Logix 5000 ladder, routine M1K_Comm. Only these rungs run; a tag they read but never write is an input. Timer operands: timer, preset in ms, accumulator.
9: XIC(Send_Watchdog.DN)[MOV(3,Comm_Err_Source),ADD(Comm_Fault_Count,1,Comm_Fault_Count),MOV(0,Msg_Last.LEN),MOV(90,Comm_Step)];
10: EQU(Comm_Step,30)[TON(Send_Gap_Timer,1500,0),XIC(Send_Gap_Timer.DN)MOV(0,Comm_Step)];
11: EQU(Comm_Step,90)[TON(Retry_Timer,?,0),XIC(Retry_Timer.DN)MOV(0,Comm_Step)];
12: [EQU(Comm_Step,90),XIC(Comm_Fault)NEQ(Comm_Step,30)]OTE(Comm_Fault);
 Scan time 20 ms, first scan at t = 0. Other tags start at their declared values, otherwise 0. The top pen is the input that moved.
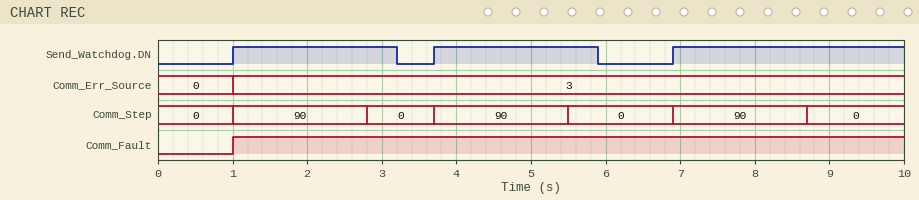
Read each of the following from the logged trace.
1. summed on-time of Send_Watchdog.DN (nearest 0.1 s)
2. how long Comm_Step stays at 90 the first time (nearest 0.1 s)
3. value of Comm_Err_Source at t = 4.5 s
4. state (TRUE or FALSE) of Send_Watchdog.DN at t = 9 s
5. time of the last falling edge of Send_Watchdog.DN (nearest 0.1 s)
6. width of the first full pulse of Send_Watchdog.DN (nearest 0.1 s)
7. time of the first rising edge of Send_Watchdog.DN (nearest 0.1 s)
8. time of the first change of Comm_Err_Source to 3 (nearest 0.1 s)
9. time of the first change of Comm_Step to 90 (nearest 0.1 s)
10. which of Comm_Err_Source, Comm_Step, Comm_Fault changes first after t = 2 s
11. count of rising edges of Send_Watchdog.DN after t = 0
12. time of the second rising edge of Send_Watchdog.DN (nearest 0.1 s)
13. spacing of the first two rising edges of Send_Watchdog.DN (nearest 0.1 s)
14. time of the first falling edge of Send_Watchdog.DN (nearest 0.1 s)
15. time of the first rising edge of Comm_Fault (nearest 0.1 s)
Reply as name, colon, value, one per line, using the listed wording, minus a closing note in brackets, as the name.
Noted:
summed on-time of Send_Watchdog.DN: 7.5 s
how long Comm_Step stays at 90 the first time: 1.8 s
value of Comm_Err_Source at t = 4.5 s: 3
state (TRUE or FALSE) of Send_Watchdog.DN at t = 9 s: TRUE
time of the last falling edge of Send_Watchdog.DN: 5.9 s
width of the first full pulse of Send_Watchdog.DN: 2.2 s
time of the first rising edge of Send_Watchdog.DN: 1.0 s
time of the first change of Comm_Err_Source to 3: 1.0 s
time of the first change of Comm_Step to 90: 1.0 s
which of Comm_Err_Source, Comm_Step, Comm_Fault changes first after t = 2 s: Comm_Step
count of rising edges of Send_Watchdog.DN after t = 0: 3
time of the second rising edge of Send_Watchdog.DN: 3.7 s
spacing of the first two rising edges of Send_Watchdog.DN: 2.7 s
time of the first falling edge of Send_Watchdog.DN: 3.2 s
time of the first rising edge of Comm_Fault: 1.0 s
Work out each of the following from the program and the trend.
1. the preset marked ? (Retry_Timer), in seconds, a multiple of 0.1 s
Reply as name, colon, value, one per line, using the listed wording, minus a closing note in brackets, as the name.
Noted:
the preset marked ? (Retry_Timer), in seconds, a multiple of 0.1 s: 1.8 s
